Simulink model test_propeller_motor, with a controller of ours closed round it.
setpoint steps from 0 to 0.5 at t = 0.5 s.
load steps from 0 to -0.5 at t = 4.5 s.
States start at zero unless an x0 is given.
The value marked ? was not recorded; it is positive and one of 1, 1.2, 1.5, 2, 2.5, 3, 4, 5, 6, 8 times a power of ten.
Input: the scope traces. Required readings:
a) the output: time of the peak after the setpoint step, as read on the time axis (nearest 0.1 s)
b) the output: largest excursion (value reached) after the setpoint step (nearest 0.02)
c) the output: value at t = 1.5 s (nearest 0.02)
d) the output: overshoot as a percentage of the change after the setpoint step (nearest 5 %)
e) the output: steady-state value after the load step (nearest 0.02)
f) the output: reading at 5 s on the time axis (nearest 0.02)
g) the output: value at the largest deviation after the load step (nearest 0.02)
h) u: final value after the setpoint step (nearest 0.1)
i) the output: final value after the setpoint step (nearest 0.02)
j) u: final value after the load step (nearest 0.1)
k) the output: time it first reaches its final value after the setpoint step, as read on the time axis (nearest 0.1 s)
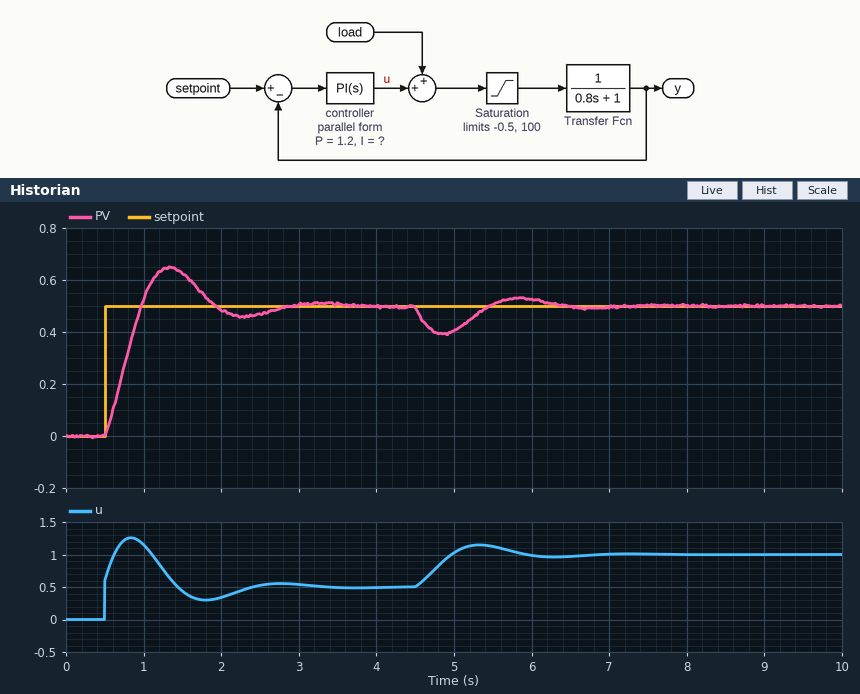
1.3 s
0.64
0.62
30 %
0.50
0.40
0.40
0.5
0.50
1.0
1.0 s
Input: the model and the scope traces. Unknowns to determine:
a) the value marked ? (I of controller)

10
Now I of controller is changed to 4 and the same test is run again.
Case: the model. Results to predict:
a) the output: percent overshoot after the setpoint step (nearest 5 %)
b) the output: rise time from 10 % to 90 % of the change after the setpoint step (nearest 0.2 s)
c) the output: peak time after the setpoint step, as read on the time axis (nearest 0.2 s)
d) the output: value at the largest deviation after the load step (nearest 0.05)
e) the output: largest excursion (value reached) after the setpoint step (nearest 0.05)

10 %
0.6 s
1.8 s
0.35
0.55
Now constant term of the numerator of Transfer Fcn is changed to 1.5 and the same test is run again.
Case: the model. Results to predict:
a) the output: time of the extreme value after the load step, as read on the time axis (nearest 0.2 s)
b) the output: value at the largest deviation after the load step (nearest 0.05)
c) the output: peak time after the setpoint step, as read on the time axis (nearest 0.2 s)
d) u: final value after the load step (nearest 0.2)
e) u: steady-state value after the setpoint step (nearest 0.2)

4.8 s
0.35
1.2 s
0.8
0.4
